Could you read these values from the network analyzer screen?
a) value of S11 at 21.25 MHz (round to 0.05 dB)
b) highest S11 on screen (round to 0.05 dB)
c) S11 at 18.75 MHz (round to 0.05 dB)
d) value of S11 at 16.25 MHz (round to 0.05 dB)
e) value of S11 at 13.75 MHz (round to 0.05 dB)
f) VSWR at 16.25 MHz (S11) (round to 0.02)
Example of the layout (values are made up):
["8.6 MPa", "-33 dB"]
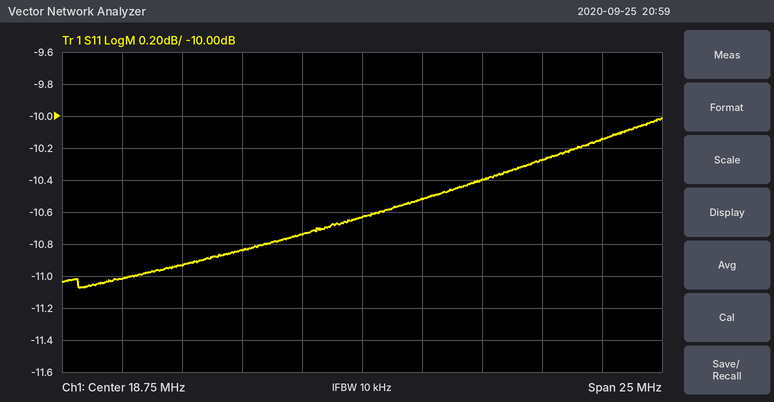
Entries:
["-10.50 dB", "-10.00 dB", "-10.65 dB", "-10.75 dB", "-10.85 dB", "1.82"]
